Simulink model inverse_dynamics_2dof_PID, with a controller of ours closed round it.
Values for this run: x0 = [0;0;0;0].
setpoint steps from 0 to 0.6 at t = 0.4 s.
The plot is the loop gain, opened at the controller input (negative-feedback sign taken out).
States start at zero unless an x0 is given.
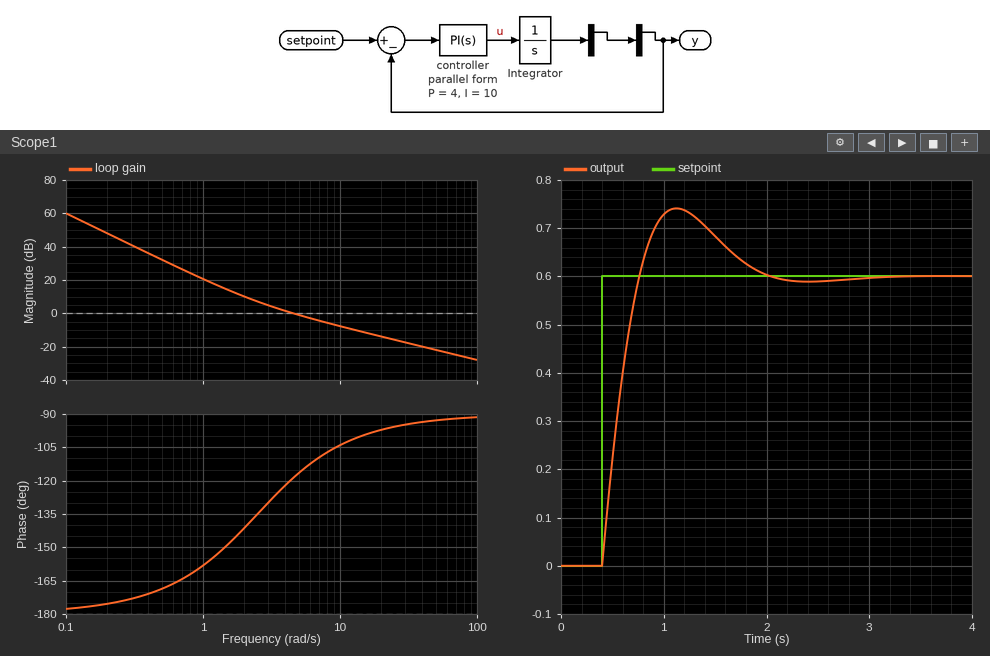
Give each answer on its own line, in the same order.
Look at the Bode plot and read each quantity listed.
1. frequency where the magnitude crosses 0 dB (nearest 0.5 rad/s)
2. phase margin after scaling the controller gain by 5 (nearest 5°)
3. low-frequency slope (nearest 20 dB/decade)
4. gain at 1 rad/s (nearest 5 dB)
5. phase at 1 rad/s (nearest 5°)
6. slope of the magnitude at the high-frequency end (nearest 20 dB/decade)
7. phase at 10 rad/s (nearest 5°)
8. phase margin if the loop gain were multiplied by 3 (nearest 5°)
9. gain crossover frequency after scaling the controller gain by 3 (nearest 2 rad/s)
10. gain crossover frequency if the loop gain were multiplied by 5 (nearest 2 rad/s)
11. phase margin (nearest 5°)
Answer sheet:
4.5 rad/s
85°
-40 dB/decade
20 dB
-160°
-20 dB/decade
-105°
80°
12 rad/s
20 rad/s
60°
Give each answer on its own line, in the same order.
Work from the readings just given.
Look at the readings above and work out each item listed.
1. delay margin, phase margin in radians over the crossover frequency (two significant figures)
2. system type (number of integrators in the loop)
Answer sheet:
0.23 s
2
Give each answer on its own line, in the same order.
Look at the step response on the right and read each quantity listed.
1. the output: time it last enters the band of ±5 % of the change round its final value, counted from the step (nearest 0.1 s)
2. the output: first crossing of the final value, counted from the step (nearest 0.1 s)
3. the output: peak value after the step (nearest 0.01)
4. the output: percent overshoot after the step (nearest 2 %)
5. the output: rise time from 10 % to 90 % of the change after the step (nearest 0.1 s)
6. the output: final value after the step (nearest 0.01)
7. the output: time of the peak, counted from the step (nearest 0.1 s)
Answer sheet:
1.4 s
0.4 s
0.74
24 %
0.3 s
0.60
0.7 s
